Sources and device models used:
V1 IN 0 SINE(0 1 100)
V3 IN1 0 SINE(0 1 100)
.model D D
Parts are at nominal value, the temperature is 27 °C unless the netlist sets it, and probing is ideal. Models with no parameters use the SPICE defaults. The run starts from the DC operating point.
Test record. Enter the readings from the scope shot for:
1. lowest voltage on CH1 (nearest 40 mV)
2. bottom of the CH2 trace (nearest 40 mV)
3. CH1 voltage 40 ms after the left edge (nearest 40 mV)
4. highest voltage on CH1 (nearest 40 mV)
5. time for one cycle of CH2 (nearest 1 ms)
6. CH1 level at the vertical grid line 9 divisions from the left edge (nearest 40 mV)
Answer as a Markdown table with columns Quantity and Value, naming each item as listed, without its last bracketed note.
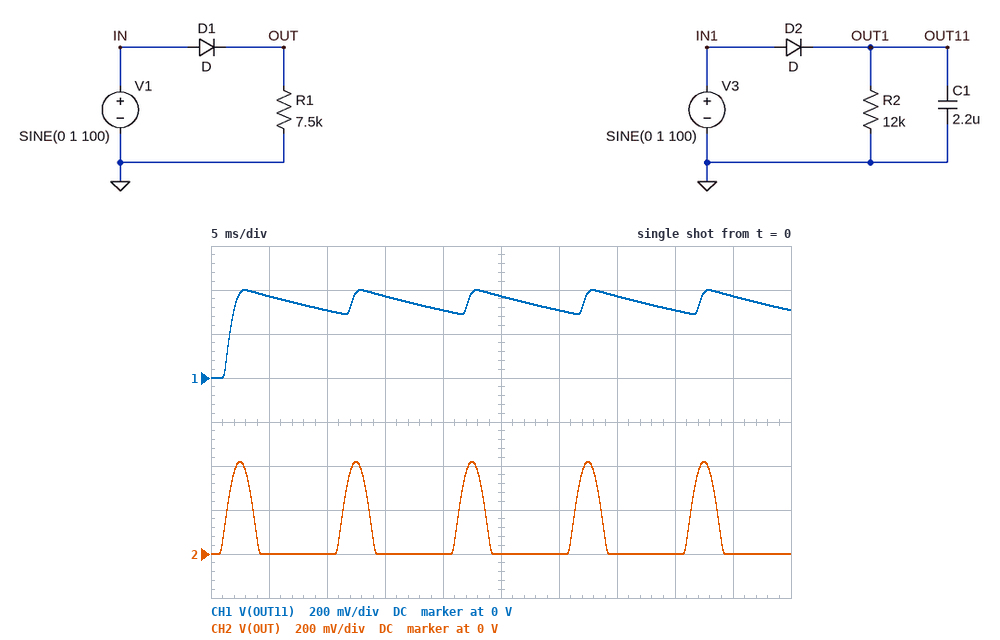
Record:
| Quantity | Value |
|---|---|
| lowest voltage on CH1 | 0 V |
| bottom of the CH2 trace | 0 V |
| CH1 voltage 40 ms after the left edge | 320 mV |
| highest voltage on CH1 | 400 mV |
| time for one cycle of CH2 | 10 ms |
| CH1 level at the vertical grid line 9 divisions from the left edge | 360 mV |
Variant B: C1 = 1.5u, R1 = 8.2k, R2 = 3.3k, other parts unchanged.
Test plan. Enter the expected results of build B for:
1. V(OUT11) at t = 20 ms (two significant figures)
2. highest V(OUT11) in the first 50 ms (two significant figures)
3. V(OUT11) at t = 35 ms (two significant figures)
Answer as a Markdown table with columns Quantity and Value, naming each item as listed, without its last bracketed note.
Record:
| Quantity | Value |
|---|---|
| V(OUT11) at t = 20 ms | 94 mV |
| highest V(OUT11) in the first 50 ms | 390 mV |
| V(OUT11) at t = 35 ms | 260 mV |
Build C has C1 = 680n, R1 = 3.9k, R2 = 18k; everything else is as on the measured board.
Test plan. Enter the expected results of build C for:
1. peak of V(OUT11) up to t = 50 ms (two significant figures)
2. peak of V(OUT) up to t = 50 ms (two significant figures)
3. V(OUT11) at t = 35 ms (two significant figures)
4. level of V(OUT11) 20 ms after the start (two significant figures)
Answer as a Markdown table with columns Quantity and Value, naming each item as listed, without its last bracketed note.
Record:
| Quantity | Value |
|---|---|
| peak of V(OUT11) up to t = 50 ms | 420 mV |
| peak of V(OUT) up to t = 50 ms | 400 mV |
| V(OUT11) at t = 35 ms | 360 mV |
| level of V(OUT11) 20 ms after the start | 240 mV |
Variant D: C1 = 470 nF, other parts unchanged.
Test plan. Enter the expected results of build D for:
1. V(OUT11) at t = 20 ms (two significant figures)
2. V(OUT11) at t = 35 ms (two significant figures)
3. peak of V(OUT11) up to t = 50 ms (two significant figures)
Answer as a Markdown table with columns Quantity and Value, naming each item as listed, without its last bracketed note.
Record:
| Quantity | Value |
|---|---|
| V(OUT11) at t = 20 ms | 120 mV |
| V(OUT11) at t = 35 ms | 290 mV |
| peak of V(OUT11) up to t = 50 ms | 420 mV |
